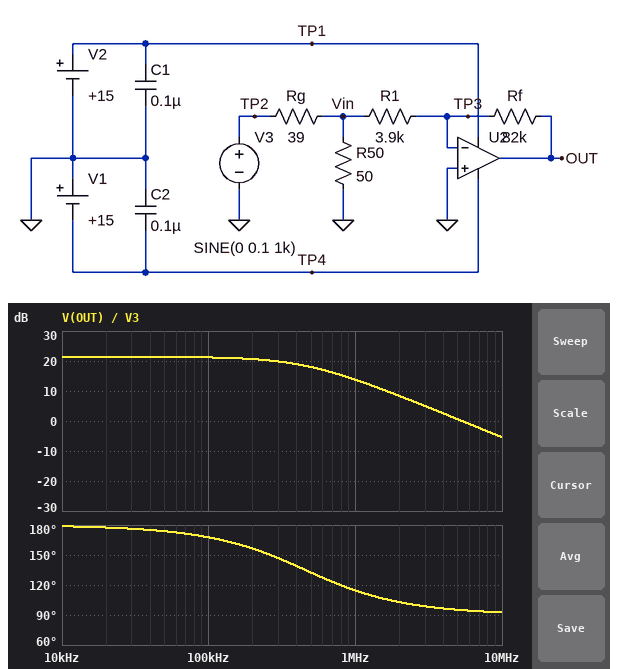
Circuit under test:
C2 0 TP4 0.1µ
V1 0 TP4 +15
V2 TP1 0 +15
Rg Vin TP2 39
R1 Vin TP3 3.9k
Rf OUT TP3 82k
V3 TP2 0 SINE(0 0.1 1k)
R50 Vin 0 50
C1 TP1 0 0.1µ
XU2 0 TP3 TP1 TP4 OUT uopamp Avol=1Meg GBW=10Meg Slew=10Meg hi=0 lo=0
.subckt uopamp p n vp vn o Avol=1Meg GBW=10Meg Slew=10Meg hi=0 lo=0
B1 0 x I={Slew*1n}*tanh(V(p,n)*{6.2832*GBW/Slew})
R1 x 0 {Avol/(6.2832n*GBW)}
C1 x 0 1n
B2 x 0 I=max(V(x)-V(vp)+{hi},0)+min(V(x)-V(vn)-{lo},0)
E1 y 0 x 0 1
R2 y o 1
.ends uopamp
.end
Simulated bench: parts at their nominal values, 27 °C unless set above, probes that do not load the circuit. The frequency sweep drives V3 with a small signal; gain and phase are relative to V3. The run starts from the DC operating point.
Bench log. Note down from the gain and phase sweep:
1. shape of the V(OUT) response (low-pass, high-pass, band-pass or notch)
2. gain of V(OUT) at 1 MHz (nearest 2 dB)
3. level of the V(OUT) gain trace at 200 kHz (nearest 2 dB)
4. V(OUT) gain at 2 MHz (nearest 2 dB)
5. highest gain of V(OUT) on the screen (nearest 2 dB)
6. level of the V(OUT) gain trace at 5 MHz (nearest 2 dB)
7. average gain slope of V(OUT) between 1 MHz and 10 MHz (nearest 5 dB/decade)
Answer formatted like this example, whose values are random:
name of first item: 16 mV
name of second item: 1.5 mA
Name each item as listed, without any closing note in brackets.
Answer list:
shape of the V(OUT) response: low-pass
gain of V(OUT) at 1 MHz: 14 dB
level of the V(OUT) gain trace at 200 kHz: 20 dB
V(OUT) gain at 2 MHz: 8 dB
highest gain of V(OUT) on the screen: 22 dB
level of the V(OUT) gain trace at 5 MHz: 0 dB
average gain slope of V(OUT) between 1 MHz and 10 MHz: -20 dB/decade
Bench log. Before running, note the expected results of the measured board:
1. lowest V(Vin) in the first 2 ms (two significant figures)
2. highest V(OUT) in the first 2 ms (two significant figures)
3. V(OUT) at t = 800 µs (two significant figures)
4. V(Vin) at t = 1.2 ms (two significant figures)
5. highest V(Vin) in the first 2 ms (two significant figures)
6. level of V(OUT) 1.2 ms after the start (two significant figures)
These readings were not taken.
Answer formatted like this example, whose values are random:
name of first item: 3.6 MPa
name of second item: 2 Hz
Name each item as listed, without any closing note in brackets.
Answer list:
lowest V(Vin) in the first 2 ms: -56 mV
highest V(OUT) in the first 2 ms: 1.2 V
V(OUT) at t = 800 µs: 1.1 V
V(Vin) at t = 1.2 ms: 53 mV
highest V(Vin) in the first 2 ms: 56 mV
level of V(OUT) 1.2 ms after the start: -1.1 V
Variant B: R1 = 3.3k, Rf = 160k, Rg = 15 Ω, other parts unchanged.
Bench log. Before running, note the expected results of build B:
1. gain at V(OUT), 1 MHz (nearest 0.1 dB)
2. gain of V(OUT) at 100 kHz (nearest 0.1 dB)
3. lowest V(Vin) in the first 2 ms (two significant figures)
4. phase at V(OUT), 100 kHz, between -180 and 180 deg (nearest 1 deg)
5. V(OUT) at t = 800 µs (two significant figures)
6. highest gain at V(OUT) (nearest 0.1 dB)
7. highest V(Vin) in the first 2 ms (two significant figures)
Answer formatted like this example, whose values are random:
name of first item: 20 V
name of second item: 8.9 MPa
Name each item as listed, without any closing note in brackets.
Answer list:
gain at V(OUT), 1 MHz: 17.4 dB
gain of V(OUT) at 100 kHz: 30.5 dB
lowest V(Vin) in the first 2 ms: -77 mV
phase at V(OUT), 100 kHz, between -180 and 180 deg: 154 deg
V(OUT) at t = 800 µs: 3.5 V
highest gain at V(OUT): 31.4 dB
highest V(Vin) in the first 2 ms: 77 mV
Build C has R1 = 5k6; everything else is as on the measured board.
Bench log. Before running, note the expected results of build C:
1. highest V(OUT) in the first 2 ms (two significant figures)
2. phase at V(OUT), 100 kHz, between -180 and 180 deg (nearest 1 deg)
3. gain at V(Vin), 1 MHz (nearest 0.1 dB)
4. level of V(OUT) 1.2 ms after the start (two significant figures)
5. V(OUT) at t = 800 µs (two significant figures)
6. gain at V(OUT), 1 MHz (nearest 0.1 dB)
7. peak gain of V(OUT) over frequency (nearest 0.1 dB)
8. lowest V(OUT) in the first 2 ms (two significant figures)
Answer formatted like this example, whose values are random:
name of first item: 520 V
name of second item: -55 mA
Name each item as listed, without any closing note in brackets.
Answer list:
highest V(OUT) in the first 2 ms: 820 mV
phase at V(OUT), 100 kHz, between -180 and 180 deg: 171 deg
gain at V(Vin), 1 MHz: -5.0 dB
level of V(OUT) 1.2 ms after the start: -780 mV
V(OUT) at t = 800 µs: 780 mV
gain at V(OUT), 1 MHz: 12.9 dB
peak gain of V(OUT) over frequency: 18.3 dB
lowest V(OUT) in the first 2 ms: -820 mV
